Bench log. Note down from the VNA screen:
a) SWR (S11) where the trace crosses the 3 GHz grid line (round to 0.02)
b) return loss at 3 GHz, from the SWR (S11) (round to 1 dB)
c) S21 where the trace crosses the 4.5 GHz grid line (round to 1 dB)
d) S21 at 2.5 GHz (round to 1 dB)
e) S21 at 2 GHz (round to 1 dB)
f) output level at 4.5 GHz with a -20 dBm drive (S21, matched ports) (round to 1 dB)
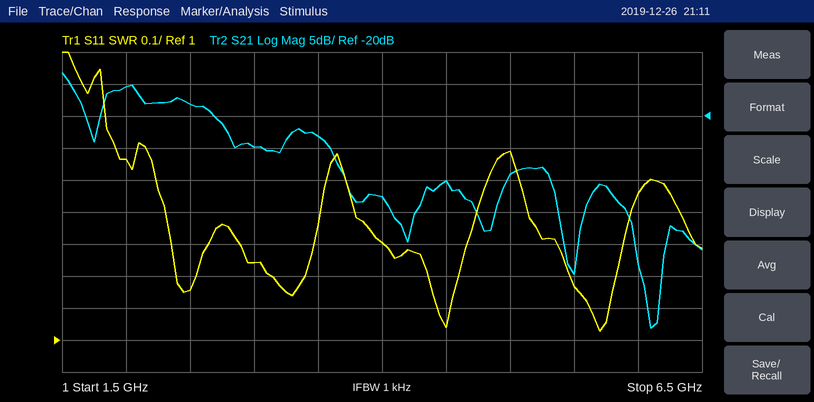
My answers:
1.24
19 dB
-30 dB
-18 dB
-15 dB
-50 dBm
